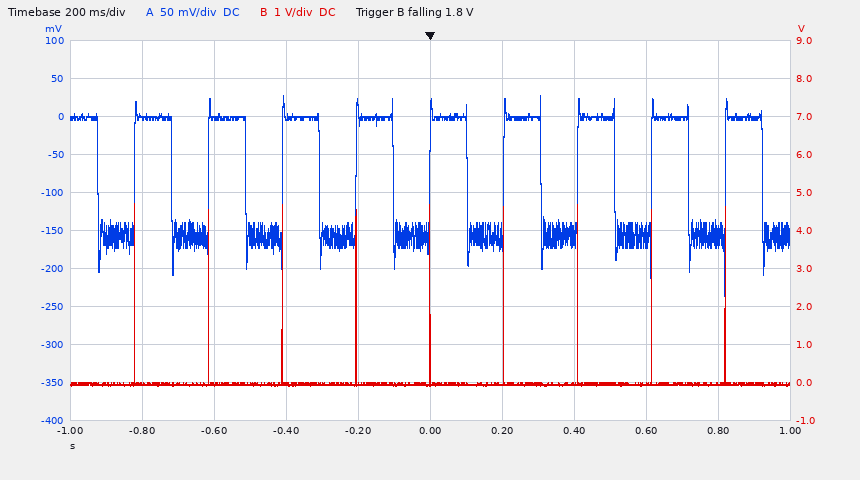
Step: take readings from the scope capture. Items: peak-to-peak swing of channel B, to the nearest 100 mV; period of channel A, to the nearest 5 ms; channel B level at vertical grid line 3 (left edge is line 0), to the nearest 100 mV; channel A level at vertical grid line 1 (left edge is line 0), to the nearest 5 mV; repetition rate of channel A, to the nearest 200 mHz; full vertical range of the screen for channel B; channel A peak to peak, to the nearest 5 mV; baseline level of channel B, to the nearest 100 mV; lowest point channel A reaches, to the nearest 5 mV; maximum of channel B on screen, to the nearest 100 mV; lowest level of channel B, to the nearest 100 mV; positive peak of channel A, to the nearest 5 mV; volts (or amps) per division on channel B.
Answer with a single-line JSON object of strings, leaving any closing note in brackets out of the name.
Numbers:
{"peak-to-peak swing of channel B, to the nearest 100 mV": "4.8 V", "period of channel A, to the nearest 5 ms": "205 ms", "channel B level at vertical grid line 3 (left edge is line 0), to the nearest 100 mV": "0.0 V", "channel A level at vertical grid line 1 (left edge is line 0), to the nearest 5 mV": "0 mV", "repetition rate of channel A, to the nearest 200 mHz": "4.8 Hz", "full vertical range of the screen for channel B": "10 V", "channel A peak to peak, to the nearest 5 mV": "265 mV", "baseline level of channel B, to the nearest 100 mV": "0.0 V", "lowest point channel A reaches, to the nearest 5 mV": "-235 mV", "maximum of channel B on screen, to the nearest 100 mV": "4.7 V", "lowest level of channel B, to the nearest 100 mV": "-100 mV", "positive peak of channel A, to the nearest 5 mV": "30 mV", "volts (or amps) per division on channel B": "1 V"}
